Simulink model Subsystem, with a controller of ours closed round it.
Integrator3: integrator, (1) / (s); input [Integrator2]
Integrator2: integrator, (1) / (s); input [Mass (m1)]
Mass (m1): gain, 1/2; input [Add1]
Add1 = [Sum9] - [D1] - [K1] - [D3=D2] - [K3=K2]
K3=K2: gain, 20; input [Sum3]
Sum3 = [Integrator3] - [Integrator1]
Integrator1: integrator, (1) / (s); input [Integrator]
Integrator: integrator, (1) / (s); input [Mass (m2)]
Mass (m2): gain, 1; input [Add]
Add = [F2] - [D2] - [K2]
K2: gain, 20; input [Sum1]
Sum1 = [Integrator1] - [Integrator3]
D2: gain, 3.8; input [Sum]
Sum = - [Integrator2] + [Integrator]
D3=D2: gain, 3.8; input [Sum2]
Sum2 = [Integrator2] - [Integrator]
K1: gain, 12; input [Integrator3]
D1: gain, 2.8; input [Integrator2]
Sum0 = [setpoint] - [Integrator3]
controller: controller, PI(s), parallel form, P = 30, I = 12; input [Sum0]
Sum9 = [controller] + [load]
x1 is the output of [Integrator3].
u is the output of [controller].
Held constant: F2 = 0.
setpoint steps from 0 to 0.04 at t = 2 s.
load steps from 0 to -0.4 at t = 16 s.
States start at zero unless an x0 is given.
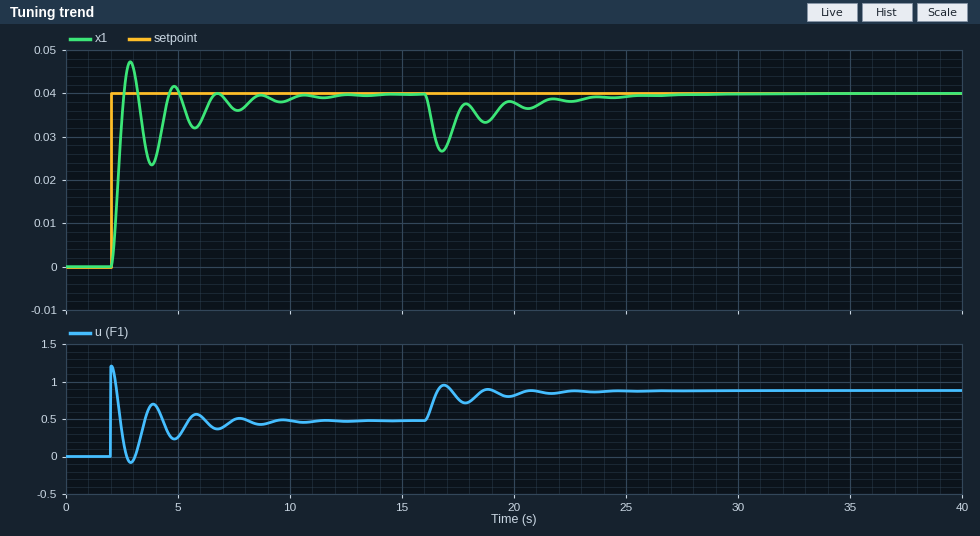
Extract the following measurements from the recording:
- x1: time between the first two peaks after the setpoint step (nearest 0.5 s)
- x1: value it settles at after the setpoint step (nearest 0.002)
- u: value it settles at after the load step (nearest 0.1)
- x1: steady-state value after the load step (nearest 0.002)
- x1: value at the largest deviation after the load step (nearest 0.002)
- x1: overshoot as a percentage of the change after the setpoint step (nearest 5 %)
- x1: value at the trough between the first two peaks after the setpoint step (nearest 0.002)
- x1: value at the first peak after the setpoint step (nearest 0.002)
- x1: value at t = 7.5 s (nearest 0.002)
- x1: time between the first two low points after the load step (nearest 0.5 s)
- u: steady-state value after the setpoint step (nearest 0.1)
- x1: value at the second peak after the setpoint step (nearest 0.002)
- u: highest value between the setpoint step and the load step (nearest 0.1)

2.0 s
0.040
0.9
0.040
0.026
20 %
0.024
0.048
0.036
2.0 s
0.5
0.042
1.2
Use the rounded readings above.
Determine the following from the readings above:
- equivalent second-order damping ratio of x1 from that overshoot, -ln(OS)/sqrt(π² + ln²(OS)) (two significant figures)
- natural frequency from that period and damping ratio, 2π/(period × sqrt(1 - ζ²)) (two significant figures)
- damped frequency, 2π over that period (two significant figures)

0.46
3.5 rad/s
3.1 rad/s
